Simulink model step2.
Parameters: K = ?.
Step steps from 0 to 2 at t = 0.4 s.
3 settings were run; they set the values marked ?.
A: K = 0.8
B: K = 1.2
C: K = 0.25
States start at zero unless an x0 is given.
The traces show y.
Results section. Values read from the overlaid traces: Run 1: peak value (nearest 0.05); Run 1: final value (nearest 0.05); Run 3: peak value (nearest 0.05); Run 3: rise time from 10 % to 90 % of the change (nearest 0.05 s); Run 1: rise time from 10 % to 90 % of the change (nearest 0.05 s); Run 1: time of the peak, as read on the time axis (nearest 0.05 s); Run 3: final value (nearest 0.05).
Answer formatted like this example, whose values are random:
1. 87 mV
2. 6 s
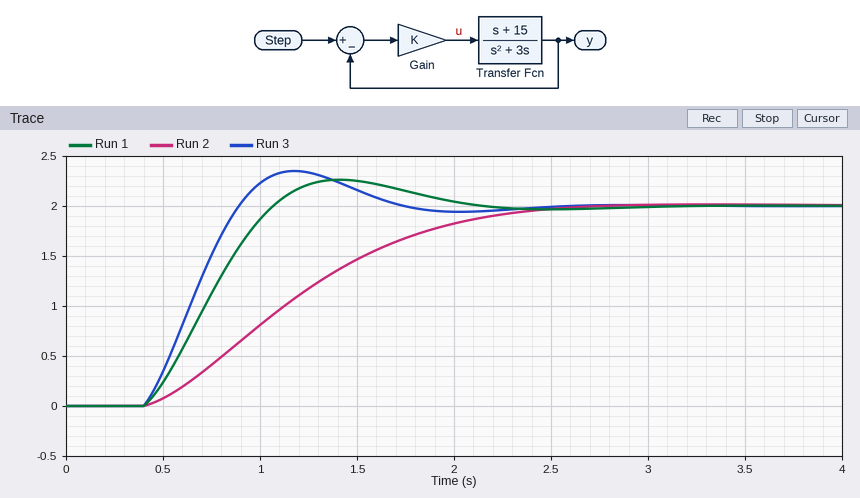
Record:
1. 2.25
2. 2.00
3. 2.35
4. 0.35 s
5. 0.50 s
6. 1.40 s
7. 2.00
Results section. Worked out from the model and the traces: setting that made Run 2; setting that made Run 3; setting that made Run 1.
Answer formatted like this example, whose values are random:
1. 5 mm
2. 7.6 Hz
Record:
1. C
2. B
3. A
